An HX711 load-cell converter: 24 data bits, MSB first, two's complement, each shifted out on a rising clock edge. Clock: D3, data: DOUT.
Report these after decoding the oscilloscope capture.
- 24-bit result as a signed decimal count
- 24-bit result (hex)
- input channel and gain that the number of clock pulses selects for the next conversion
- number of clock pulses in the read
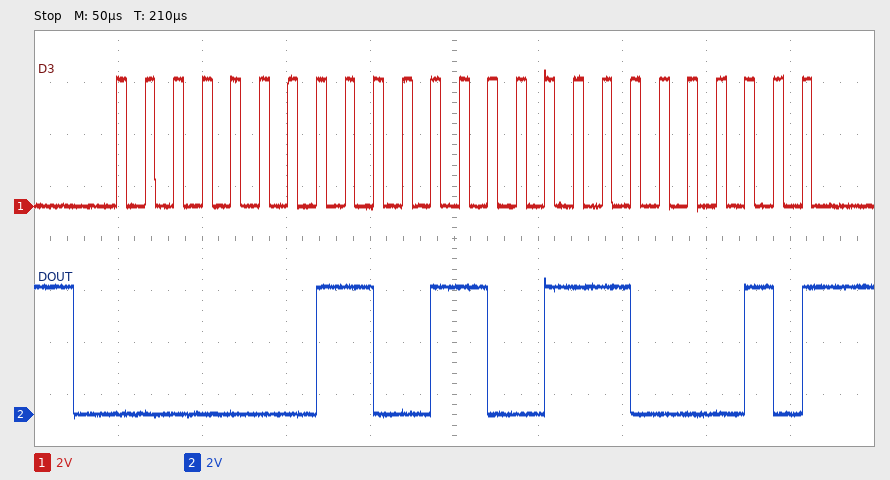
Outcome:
104898
0x0199C2
channel A, gain 128
25
